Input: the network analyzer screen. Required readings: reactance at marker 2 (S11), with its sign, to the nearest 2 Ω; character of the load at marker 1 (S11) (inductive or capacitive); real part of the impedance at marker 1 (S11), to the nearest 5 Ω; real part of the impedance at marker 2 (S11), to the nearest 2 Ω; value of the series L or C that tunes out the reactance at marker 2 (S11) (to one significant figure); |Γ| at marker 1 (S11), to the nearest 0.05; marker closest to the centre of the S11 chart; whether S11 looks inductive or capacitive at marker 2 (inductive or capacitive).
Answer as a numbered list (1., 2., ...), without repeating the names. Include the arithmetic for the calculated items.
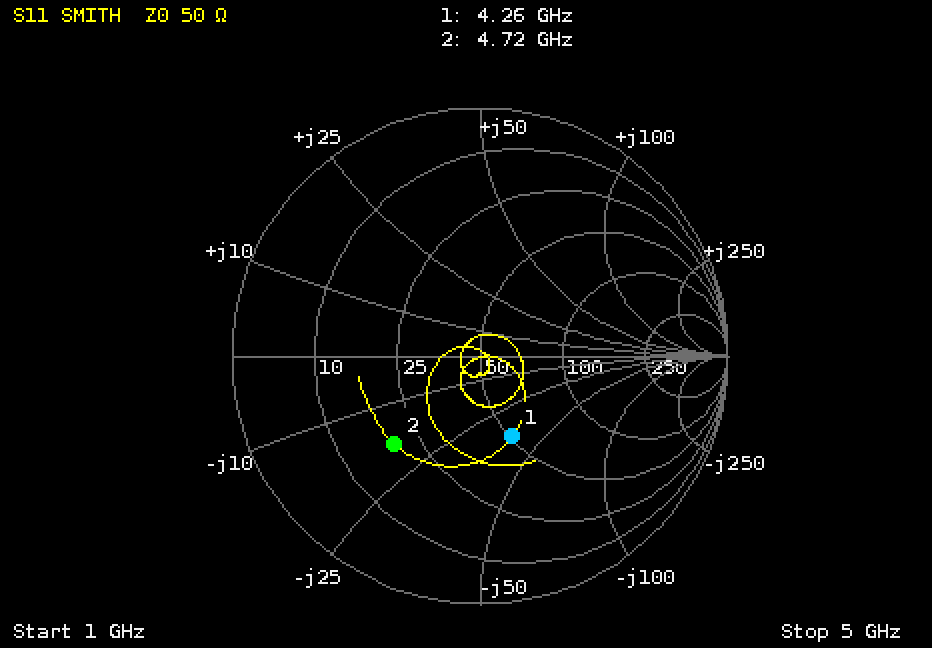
1. -18 Ω
2. capacitive
3. 50 Ω
4. 20 Ω
5. L = 18 Ω/(2π × 4.72 GHz) ≈ 607 pH, so 600 pH to one significant figure
6. 0.35
7. marker 1
8. capacitive
